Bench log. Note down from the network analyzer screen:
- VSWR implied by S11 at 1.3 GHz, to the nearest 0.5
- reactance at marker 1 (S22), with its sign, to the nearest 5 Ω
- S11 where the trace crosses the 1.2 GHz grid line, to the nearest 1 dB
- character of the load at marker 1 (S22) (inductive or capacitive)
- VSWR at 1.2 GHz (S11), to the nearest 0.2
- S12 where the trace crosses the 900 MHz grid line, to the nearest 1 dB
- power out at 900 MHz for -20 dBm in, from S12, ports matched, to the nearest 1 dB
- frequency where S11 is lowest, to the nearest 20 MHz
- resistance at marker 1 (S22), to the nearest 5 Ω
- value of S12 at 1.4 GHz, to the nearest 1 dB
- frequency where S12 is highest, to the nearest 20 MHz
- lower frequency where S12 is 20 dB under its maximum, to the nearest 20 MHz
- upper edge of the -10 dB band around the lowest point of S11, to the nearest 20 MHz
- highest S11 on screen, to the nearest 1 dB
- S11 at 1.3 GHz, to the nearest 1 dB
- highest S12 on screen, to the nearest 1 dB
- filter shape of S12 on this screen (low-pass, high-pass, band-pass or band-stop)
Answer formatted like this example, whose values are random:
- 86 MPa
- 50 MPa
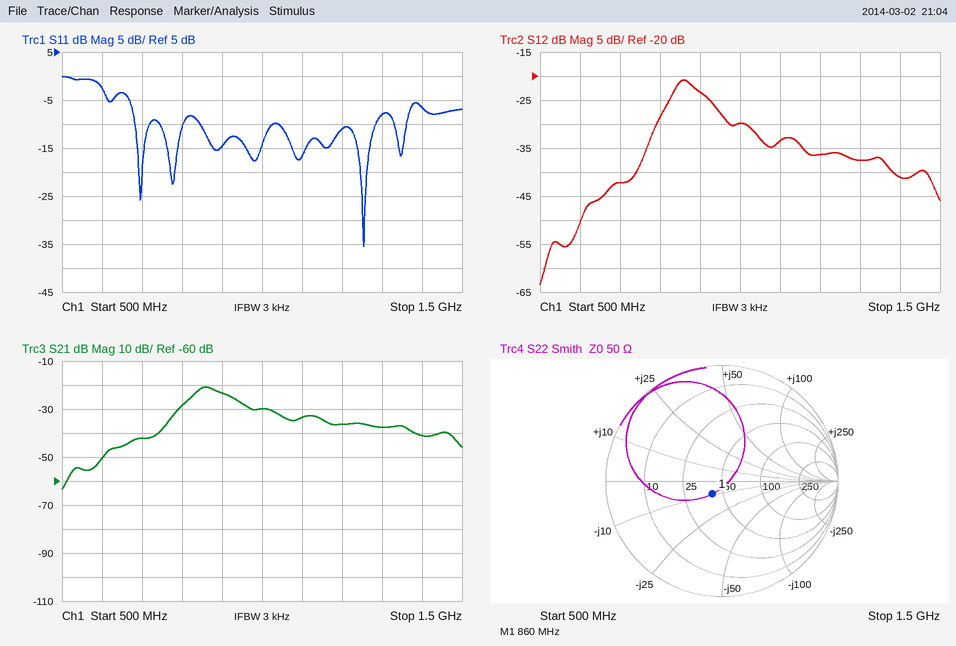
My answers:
- 2.5
- -10 Ω
- -11 dB
- capacitive
- 1.8
- -23 dB
- -43 dBm
- 1.26 GHz
- 40 Ω
- -41 dB
- 860 MHz
- 740 MHz
- 1.28 GHz
- 0 dB
- -8 dB
- -21 dB
- band-pass
